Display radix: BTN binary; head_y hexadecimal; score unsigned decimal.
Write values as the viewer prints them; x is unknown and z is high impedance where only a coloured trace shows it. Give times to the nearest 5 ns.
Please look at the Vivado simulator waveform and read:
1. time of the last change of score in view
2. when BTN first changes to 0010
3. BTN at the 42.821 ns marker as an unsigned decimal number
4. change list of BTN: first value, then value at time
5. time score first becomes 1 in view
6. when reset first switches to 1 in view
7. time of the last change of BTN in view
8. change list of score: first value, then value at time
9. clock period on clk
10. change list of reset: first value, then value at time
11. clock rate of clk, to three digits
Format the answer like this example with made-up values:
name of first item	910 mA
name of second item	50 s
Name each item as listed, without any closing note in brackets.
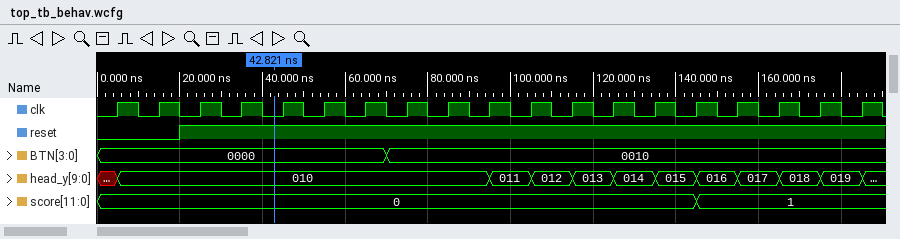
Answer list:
time of the last change of score in view	145 ns
when BTN first changes to 0010	70 ns
BTN at the 42.821 ns marker as an unsigned decimal number	0
change list of BTN: first value, then value at time	0000, 0010 at 70 ns
time score first becomes 1 in view	145 ns
when reset first switches to 1 in view	20 ns
time of the last change of BTN in view	70 ns
change list of score: first value, then value at time	0, 1 at 145 ns
clock period on clk	10 ns
change list of reset: first value, then value at time	0, 1 at 20 ns
clock rate of clk, to three digits	100 MHz
